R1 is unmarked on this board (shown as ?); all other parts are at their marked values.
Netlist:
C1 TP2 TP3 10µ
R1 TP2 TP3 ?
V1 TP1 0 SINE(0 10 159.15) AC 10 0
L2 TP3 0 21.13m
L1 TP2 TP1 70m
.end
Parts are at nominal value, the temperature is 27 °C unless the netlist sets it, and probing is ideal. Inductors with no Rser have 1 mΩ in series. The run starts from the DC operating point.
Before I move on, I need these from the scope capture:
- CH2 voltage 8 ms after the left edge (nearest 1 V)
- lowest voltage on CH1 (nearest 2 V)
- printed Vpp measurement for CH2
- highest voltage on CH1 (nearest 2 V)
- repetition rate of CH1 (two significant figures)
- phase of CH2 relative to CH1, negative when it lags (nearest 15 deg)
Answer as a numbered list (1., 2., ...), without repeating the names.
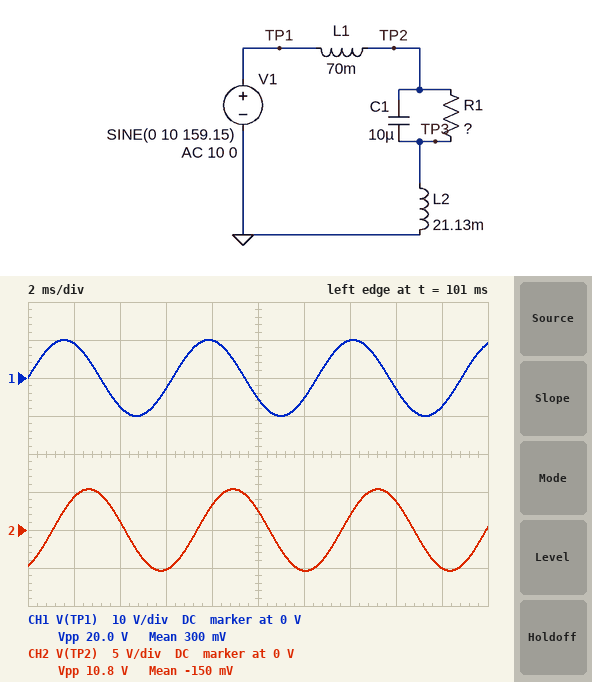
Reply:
1. 3 V
2. -10 V
3. 10.8 V
4. 10 V
5. 160 Hz
6. -60 deg
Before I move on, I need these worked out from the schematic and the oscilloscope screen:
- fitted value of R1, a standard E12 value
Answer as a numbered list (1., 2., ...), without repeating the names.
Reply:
1. 56 Ω
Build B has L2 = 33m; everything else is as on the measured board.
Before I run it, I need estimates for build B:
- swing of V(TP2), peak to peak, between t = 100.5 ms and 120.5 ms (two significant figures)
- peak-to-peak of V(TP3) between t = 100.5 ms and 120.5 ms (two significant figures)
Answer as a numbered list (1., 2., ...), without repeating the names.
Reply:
1. 9.7 V
2. 7.3 V
